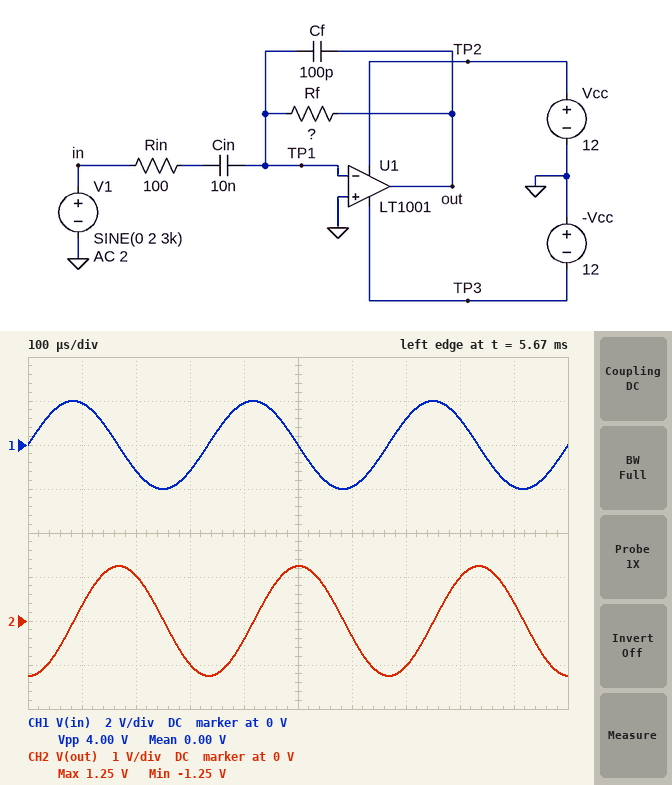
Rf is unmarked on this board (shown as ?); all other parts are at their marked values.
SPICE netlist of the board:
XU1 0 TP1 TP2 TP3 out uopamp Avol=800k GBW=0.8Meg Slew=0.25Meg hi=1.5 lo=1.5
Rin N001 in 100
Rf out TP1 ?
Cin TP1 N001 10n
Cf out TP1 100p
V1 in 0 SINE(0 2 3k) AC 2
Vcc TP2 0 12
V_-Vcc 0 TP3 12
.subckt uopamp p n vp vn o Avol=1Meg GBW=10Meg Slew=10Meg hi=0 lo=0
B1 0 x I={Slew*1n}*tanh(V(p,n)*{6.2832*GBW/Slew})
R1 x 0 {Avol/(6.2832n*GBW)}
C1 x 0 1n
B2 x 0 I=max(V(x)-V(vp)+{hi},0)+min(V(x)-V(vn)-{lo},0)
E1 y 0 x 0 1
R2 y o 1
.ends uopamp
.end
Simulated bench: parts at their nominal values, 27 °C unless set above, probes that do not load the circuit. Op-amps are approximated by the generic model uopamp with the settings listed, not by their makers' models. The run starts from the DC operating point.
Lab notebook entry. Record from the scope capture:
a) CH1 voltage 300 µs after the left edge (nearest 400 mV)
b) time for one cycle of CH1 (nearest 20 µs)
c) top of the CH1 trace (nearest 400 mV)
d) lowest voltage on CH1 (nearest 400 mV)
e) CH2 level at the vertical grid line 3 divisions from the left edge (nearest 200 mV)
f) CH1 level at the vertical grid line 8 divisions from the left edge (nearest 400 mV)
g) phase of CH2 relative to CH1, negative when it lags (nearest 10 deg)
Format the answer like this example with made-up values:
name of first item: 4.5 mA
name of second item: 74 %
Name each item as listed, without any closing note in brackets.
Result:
CH1 voltage 300 µs after the left edge: -1.2 V
time for one cycle of CH1: 340 µs
top of the CH1 trace: 2.0 V
lowest voltage on CH1: -2.0 V
CH2 level at the vertical grid line 3 divisions from the left edge: -1.0 V
CH1 level at the vertical grid line 8 divisions from the left edge: 1.2 V
phase of CH2 relative to CH1, negative when it lags: -90 deg
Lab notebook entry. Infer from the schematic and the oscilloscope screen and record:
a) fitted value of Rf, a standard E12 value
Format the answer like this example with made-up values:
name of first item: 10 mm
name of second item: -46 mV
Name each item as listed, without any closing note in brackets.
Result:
fitted value of Rf, a standard E12 value: 3.3 kΩ
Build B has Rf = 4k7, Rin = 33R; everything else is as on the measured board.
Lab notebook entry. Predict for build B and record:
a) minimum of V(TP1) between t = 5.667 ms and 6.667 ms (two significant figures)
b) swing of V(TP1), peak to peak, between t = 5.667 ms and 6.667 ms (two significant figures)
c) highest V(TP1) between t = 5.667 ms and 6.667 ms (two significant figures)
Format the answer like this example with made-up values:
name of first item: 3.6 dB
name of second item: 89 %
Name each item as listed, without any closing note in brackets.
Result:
minimum of V(TP1) between t = 5.667 ms and 6.667 ms: -6.7 mV
swing of V(TP1), peak to peak, between t = 5.667 ms and 6.667 ms: 13 mV
highest V(TP1) between t = 5.667 ms and 6.667 ms: 6.7 mV
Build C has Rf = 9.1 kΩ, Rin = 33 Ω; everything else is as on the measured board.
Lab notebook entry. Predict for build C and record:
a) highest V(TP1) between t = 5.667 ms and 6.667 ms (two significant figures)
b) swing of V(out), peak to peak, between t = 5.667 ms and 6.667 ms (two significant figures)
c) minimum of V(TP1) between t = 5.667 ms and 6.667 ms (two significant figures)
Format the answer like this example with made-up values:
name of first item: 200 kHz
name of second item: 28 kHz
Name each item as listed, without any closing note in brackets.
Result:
highest V(TP1) between t = 5.667 ms and 6.667 ms: 13 mV
swing of V(out), peak to peak, between t = 5.667 ms and 6.667 ms: 6.9 V
minimum of V(TP1) between t = 5.667 ms and 6.667 ms: -13 mV
